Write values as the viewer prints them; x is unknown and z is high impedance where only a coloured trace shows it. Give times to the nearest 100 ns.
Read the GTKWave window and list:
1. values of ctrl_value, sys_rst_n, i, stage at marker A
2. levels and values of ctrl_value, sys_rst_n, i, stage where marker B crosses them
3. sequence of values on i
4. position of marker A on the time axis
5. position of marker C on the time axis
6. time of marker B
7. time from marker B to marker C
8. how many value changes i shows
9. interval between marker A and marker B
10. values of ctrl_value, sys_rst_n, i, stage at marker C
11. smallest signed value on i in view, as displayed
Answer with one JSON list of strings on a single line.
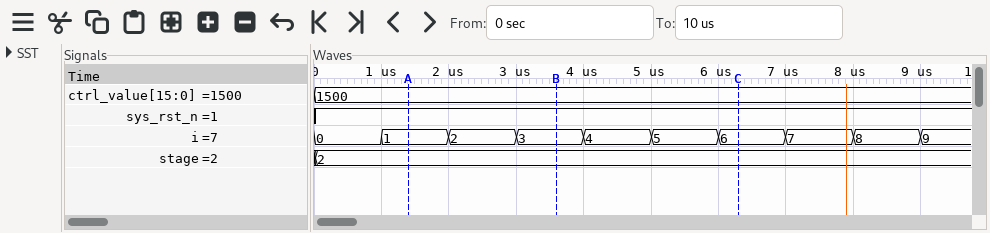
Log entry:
["ctrl_value=1500, sys_rst_n=1, i=1, stage=2", "ctrl_value=1500, sys_rst_n=1, i=3, stage=2", "0, 1, 2, 3, 4, 5, 6, 7, 8, 9", "1400 ns", "6300 ns", "3600 ns", "2700 ns", "9", "2200 ns", "ctrl_value=1500, sys_rst_n=1, i=6, stage=2", "0"]
